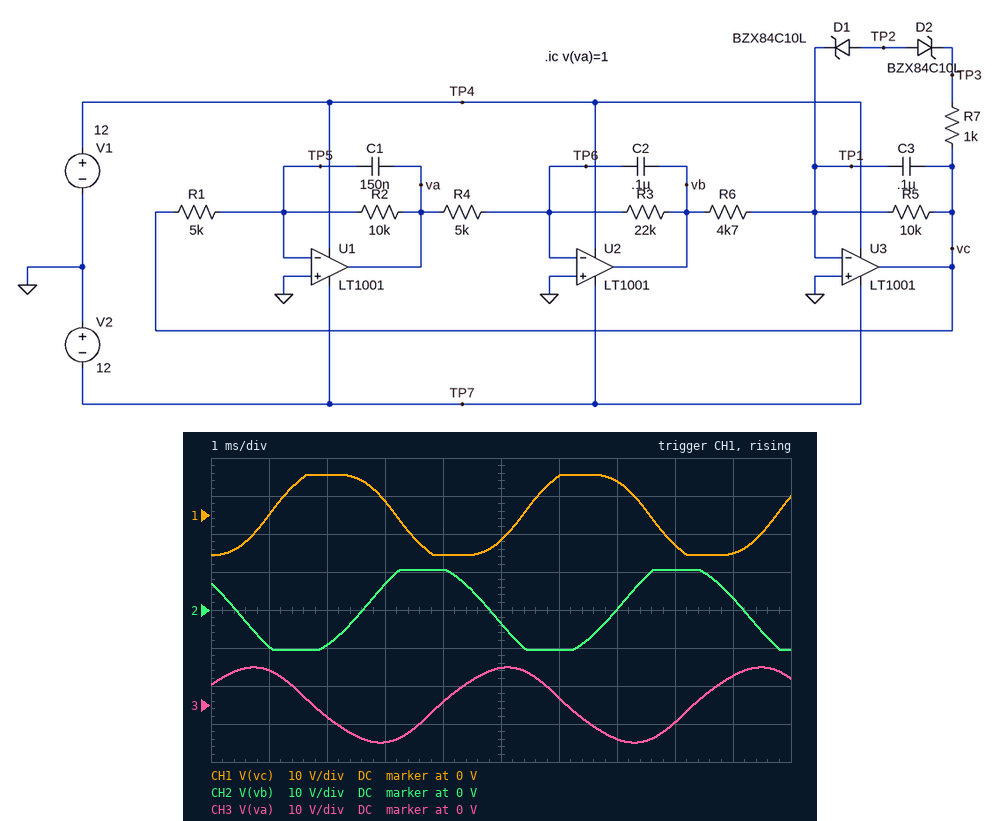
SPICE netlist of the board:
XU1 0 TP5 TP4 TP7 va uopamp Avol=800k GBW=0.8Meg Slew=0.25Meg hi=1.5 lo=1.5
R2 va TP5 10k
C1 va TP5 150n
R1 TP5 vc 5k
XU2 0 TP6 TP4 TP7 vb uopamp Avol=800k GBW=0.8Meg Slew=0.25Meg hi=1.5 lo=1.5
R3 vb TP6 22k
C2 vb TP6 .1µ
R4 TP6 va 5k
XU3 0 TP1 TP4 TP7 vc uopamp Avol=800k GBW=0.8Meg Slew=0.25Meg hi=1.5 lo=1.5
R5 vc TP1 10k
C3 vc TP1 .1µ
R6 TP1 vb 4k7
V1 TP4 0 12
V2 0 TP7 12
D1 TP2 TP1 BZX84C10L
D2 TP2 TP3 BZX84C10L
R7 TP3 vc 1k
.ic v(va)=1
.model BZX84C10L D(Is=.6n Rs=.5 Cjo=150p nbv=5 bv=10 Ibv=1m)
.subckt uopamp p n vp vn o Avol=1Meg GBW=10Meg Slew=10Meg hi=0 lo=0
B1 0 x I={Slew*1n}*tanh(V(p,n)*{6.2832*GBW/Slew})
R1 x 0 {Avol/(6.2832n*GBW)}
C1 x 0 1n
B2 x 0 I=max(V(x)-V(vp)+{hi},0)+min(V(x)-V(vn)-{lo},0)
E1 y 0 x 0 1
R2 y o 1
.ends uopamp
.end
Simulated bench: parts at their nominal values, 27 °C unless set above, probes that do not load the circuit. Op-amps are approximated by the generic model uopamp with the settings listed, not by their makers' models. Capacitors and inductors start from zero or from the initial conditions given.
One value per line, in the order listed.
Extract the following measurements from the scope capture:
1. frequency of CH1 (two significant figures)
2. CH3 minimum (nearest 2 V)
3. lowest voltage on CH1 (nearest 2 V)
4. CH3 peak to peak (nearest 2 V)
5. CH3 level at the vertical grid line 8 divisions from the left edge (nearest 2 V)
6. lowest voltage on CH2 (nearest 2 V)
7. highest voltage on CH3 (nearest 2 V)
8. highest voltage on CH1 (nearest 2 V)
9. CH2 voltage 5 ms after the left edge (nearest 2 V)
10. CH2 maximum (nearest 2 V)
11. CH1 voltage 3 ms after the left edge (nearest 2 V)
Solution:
230 Hz
-10 V
-10 V
20 V
-4 V
-10 V
10 V
10 V
-4 V
10 V
4 V
